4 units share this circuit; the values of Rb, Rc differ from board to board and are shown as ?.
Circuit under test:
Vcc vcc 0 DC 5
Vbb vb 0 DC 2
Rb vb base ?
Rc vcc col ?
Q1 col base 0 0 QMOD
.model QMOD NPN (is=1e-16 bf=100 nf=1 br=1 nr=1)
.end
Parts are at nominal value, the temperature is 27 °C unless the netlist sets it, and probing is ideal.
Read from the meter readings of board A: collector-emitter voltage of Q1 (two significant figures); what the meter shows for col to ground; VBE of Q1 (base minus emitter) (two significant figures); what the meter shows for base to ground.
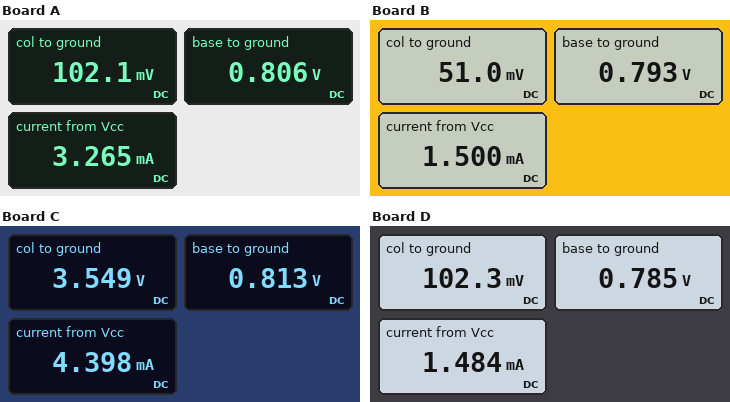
100 mV
102.1 mV
810 mV
0.806 V
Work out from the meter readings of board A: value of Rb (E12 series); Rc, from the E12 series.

12 kΩ
1.5 kΩ
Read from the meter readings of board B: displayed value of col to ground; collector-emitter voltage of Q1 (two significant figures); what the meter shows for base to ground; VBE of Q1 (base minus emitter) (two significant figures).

51.0 mV
51 mV
0.793 V
790 mV
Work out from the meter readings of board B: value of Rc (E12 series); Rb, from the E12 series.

3.3 kΩ
3.9 kΩ
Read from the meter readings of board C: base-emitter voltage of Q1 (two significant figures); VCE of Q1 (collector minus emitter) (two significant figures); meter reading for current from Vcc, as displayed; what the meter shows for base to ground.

810 mV
3.5 V
4.398 mA
0.813 V
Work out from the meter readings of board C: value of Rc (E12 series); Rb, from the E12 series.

330 Ω
27 kΩ
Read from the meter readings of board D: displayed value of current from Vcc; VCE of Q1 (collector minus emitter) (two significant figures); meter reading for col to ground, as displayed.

1.484 mA
100 mV
102.3 mV
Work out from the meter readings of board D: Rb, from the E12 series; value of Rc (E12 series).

27 kΩ
3.3 kΩ
